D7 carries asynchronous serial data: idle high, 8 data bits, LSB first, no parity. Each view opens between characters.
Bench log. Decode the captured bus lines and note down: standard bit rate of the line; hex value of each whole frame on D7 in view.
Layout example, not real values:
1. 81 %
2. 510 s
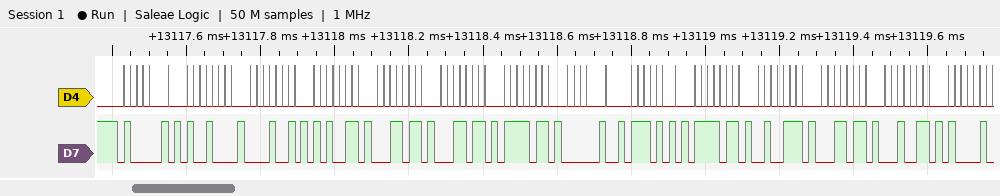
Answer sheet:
1. 57600 baud
2. 41, 09, 48, 65, 6C, 6C, 6F, 20, 57, 6F, 72, 6C, 64
